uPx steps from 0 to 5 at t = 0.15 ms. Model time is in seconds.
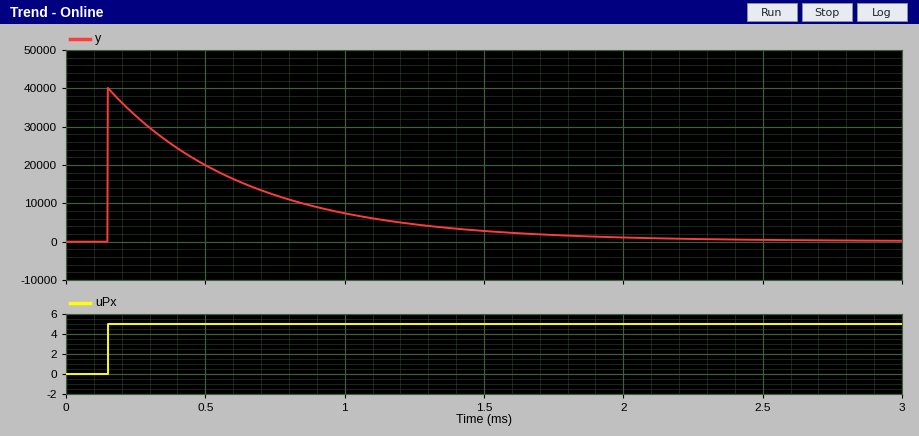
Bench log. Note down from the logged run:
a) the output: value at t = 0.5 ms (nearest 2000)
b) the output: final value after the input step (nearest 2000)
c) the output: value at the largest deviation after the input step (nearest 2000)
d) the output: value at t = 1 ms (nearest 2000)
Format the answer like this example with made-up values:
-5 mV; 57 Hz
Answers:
20000; 0; 40000; 8000
